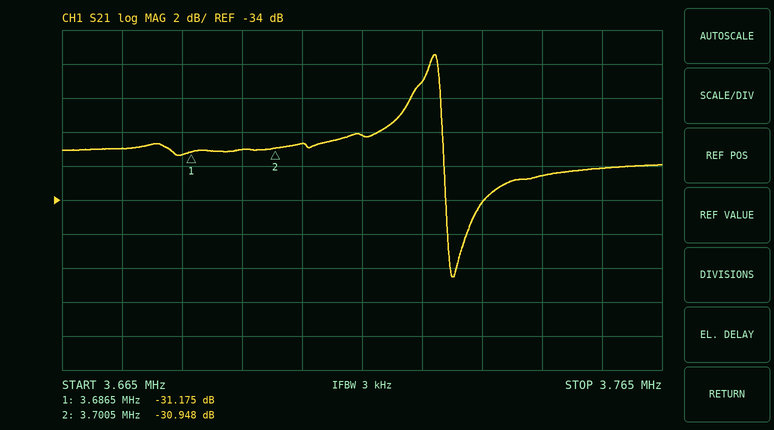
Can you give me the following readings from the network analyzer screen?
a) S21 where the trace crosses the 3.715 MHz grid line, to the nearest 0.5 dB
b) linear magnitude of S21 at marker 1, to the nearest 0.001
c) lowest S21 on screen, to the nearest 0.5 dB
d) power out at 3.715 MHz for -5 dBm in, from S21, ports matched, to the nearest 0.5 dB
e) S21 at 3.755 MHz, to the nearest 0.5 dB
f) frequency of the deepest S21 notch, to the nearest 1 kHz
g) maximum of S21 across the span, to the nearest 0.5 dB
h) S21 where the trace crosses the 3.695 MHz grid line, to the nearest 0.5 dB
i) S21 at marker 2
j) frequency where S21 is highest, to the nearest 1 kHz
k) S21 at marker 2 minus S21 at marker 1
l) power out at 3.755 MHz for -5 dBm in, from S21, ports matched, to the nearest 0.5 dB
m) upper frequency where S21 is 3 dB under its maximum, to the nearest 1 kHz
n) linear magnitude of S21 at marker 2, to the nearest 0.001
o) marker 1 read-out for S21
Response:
-30.0 dB
0.028
-38.5 dB
-35.0 dBm
-32.0 dB
3.730 MHz
-25.5 dB
-31.0 dB
-30.948 dB
3.727 MHz
0.227 dB
-37.0 dBm
3.728 MHz
0.028
-31.175 dB
